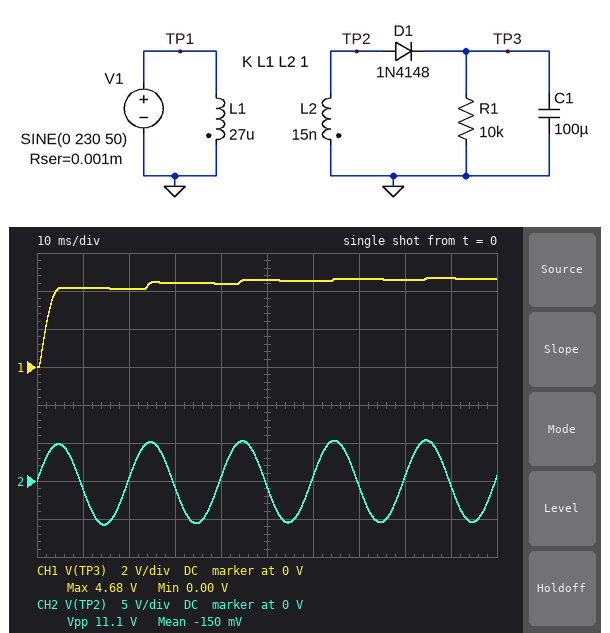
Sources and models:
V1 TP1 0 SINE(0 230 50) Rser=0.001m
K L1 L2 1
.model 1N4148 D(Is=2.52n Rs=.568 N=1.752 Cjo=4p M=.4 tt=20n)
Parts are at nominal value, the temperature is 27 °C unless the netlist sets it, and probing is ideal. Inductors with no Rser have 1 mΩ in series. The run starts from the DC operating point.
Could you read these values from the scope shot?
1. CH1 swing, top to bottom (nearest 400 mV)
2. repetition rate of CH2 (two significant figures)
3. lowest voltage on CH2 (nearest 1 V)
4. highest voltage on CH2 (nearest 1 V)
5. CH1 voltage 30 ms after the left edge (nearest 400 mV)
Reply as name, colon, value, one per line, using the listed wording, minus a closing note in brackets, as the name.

CH1 swing, top to bottom: 4.8 V
repetition rate of CH2: 50 Hz
lowest voltage on CH2: -6 V
highest voltage on CH2: 5 V
CH1 voltage 30 ms after the left edge: 4.4 V
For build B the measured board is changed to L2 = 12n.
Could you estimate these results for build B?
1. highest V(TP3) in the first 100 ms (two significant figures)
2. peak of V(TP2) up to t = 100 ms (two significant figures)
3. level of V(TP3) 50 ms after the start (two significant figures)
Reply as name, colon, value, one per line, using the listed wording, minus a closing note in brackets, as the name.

highest V(TP3) in the first 100 ms: 4.1 V
peak of V(TP2) up to t = 100 ms: 4.8 V
level of V(TP3) 50 ms after the start: 4.0 V
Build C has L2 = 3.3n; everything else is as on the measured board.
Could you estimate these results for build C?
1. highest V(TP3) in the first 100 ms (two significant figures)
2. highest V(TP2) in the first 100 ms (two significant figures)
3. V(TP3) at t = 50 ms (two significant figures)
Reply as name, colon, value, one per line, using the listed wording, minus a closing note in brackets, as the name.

highest V(TP3) in the first 100 ms: 1.9 V
highest V(TP2) in the first 100 ms: 2.5 V
V(TP3) at t = 50 ms: 1.8 V
